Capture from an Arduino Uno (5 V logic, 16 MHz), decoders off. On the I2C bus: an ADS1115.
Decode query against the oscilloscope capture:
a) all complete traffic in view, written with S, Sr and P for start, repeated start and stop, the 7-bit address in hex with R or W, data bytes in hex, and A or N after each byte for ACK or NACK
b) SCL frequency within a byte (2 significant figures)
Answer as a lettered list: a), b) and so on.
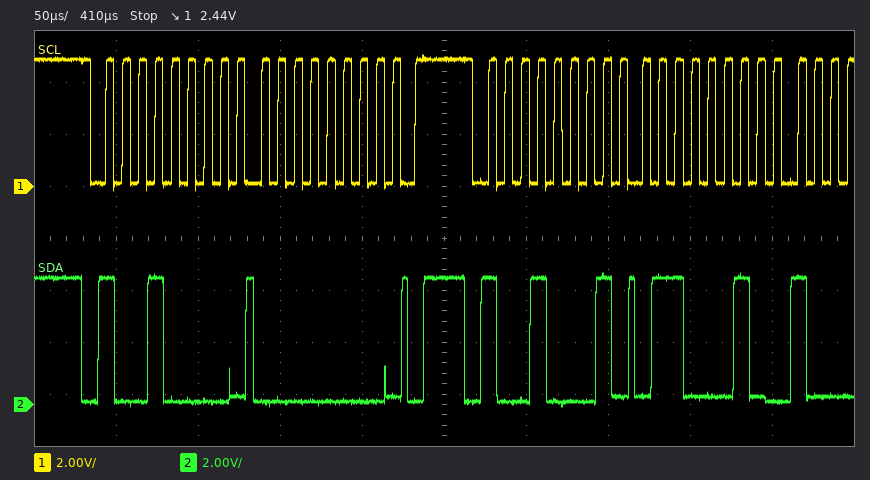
a) S 48W A 00 A P S 48R A 62 A
b) 100 kHz
